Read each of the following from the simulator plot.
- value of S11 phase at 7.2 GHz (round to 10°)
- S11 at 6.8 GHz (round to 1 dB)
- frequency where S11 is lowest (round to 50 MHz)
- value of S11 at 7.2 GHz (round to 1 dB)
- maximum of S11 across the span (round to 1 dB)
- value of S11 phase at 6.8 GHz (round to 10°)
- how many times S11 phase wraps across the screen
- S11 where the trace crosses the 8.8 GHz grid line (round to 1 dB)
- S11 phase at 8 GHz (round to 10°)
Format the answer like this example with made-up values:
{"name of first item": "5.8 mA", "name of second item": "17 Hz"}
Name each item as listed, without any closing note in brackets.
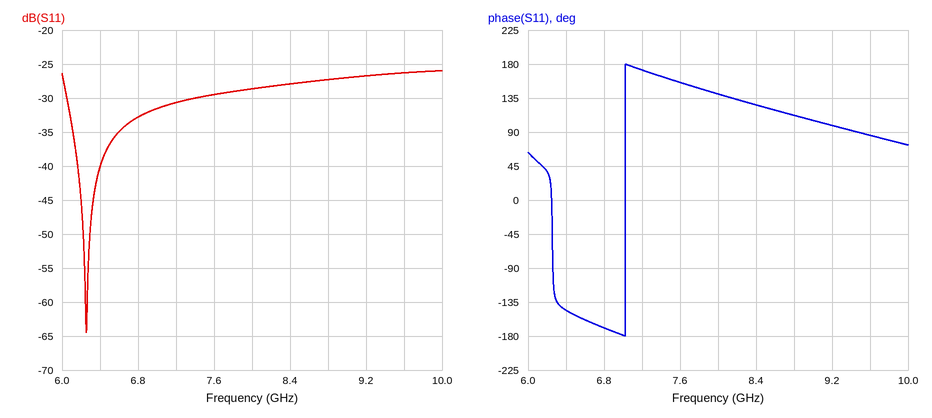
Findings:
{"value of S11 phase at 7.2 GHz": "170°", "S11 at 6.8 GHz": "-33 dB", "frequency where S11 is lowest": "6.25 GHz", "value of S11 at 7.2 GHz": "-31 dB", "maximum of S11 across the span": "-26 dB", "value of S11 phase at 6.8 GHz": "-170°", "how many times S11 phase wraps across the screen": "1", "S11 where the trace crosses the 8.8 GHz grid line": "-27 dB", "S11 phase at 8 GHz": "140°"}
